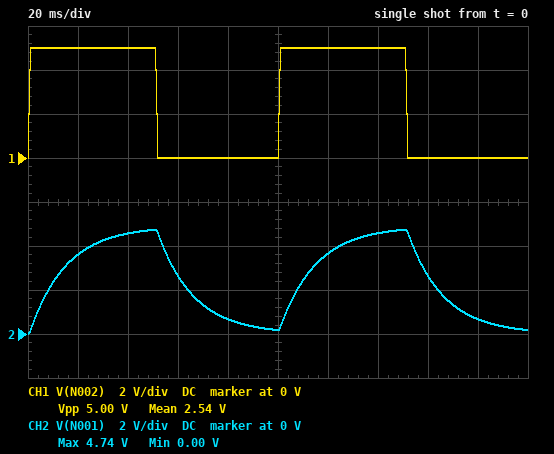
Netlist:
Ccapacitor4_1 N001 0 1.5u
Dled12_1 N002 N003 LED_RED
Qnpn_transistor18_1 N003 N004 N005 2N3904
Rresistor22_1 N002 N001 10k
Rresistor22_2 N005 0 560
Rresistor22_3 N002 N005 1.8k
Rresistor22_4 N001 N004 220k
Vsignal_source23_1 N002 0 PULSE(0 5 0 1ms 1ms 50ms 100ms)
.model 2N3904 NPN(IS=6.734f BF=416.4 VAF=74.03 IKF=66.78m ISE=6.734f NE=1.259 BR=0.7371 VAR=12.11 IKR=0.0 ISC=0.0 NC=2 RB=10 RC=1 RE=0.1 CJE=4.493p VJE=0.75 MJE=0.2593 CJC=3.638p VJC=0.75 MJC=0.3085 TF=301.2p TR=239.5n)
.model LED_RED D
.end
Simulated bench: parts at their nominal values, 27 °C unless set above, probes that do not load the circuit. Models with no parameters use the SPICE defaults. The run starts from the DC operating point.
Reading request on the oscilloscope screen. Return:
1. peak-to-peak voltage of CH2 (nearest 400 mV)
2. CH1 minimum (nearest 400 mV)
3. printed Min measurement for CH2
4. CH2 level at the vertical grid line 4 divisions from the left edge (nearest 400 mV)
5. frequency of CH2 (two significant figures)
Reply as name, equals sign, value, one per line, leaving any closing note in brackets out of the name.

peak-to-peak voltage of CH2 = 4.8 V
CH1 minimum = 0 V
printed Min measurement for CH2 = 0.00 V
CH2 level at the vertical grid line 4 divisions from the left edge = 800 mV
frequency of CH2 = 10 Hz
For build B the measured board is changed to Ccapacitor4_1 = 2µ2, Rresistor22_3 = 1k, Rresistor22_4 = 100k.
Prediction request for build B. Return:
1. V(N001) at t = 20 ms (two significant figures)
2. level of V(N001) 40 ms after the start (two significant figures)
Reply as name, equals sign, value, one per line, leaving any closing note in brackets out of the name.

V(N001) at t = 20 ms = 2.9 V
level of V(N001) 40 ms after the start = 4.1 V
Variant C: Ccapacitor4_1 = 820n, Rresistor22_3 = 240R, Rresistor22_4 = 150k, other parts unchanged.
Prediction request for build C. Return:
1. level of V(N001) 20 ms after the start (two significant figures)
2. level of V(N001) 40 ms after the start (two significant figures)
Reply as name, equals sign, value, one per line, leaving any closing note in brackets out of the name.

level of V(N001) 20 ms after the start = 4.5 V
level of V(N001) 40 ms after the start = 4.9 V
